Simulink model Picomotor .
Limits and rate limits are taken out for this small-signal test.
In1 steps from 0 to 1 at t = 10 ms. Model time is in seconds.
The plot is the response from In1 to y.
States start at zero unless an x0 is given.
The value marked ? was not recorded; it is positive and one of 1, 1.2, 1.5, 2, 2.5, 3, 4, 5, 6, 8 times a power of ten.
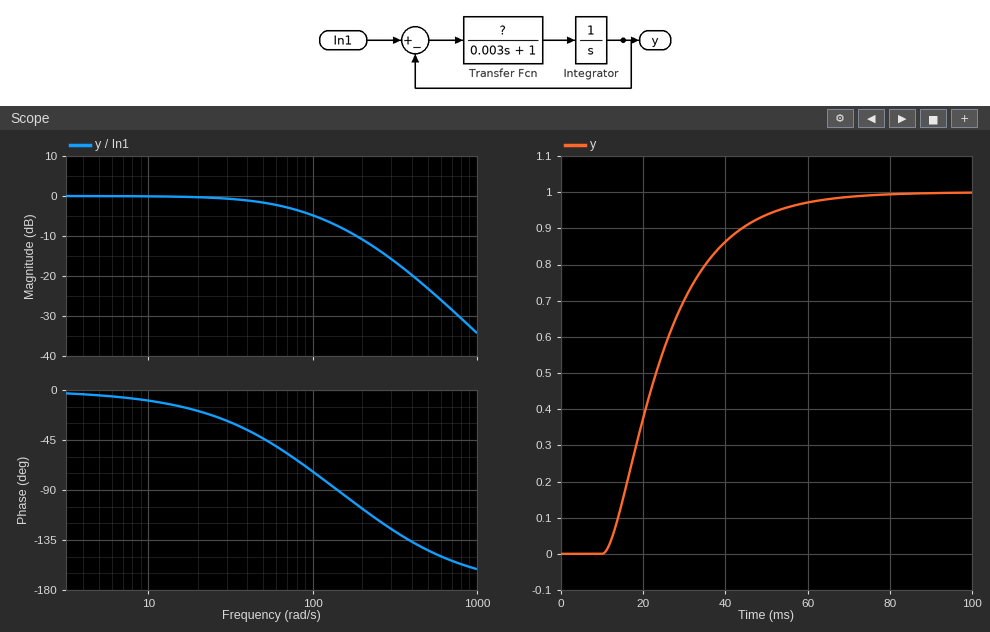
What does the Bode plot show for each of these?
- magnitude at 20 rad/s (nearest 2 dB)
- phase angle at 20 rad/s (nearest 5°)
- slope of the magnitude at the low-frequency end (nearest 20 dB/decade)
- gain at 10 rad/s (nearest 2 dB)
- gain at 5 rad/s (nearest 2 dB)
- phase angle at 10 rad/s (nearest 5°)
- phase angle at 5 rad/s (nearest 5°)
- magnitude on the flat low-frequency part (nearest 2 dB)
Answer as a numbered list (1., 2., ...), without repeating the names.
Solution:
1. 0 dB
2. -20°
3. 0 dB/decade
4. 0 dB
5. 0 dB
6. -10°
7. -5°
8. 0 dB
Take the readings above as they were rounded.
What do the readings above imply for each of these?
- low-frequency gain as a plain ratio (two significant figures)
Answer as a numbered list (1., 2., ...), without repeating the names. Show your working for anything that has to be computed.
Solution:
1. 10^(0 / 20) = 1.0
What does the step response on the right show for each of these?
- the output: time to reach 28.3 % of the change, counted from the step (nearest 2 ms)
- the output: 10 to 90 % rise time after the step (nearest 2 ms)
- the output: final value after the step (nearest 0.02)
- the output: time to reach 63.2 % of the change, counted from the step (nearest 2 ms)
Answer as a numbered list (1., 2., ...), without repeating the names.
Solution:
1. 8 ms
2. 30 ms
3. 1.00
4. 18 ms
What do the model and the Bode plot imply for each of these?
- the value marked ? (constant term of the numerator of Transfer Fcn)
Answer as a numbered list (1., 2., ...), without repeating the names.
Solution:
1. 60
